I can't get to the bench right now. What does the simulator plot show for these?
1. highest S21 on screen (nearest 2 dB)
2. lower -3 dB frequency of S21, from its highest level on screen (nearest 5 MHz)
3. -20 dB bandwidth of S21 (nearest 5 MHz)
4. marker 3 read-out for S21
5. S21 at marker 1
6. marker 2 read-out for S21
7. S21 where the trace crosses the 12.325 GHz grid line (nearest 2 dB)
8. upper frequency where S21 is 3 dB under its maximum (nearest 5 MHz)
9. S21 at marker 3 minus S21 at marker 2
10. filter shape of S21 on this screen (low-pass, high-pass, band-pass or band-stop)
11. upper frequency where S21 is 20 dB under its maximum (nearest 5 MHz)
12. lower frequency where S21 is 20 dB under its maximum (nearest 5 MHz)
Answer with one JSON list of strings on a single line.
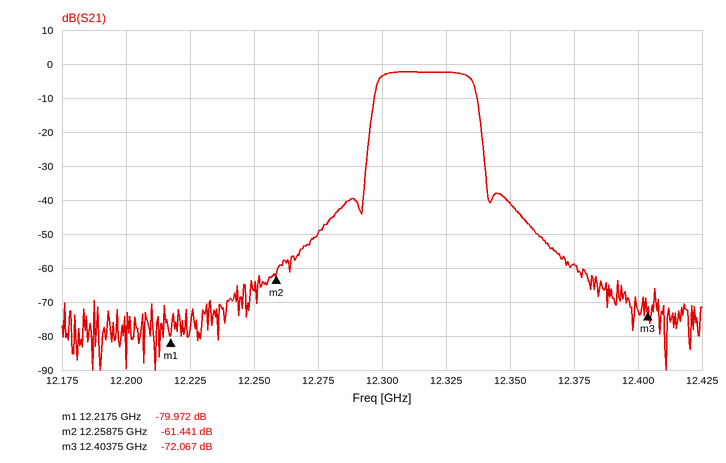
["-2 dB", "12.300 GHz", "45 MHz", "-72.067 dB", "-79.972 dB", "-61.441 dB", "-2 dB", "12.335 GHz", "-10.626 dB", "band-pass", "12.340 GHz", "12.295 GHz"]
